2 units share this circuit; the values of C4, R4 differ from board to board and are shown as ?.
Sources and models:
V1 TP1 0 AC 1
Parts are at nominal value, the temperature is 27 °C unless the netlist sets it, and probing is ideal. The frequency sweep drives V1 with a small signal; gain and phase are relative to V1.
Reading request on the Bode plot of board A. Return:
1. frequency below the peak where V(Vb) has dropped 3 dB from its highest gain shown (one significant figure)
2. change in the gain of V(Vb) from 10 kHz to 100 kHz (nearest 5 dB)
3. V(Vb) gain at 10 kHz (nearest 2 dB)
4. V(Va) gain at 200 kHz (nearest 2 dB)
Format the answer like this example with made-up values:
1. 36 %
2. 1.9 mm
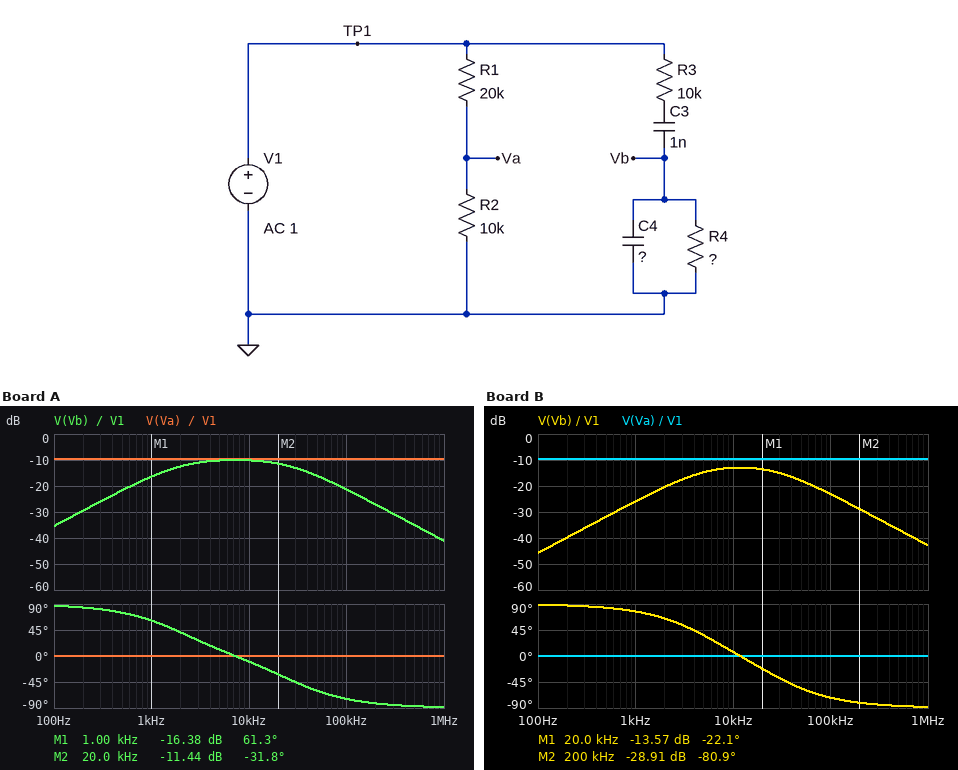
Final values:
1. 2 kHz
2. -10 dB
3. -10 dB
4. -10 dB
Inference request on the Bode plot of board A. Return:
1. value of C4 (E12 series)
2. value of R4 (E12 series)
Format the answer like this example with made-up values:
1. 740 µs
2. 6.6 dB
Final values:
1. 1.8 nF
2. 27 kΩ
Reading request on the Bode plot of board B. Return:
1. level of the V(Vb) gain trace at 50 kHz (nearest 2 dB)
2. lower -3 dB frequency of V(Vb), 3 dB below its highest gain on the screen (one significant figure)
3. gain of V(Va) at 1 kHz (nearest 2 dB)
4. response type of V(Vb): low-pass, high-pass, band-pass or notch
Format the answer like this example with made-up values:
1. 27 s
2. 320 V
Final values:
1. -18 dB
2. 4 kHz
3. -10 dB
4. band-pass
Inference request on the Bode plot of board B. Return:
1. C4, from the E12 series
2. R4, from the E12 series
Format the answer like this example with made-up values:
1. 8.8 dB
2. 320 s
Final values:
1. 2.2 nF
2. 8.2 kΩ
